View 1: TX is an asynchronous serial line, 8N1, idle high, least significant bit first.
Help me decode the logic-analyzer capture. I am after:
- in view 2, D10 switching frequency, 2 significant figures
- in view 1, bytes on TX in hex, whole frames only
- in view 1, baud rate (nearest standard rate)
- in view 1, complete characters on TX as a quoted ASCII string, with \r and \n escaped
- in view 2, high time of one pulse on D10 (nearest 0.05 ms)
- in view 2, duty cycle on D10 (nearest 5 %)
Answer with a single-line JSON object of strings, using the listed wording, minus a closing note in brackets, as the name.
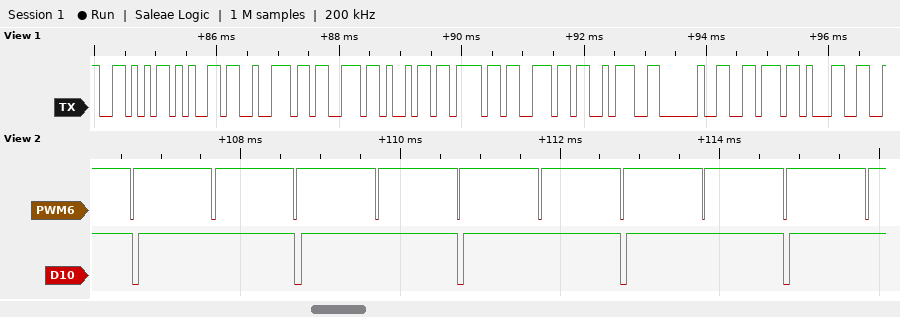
{"in view 2, D10 switching frequency, 2 significant figures": "490 Hz", "in view 1, bytes on TX in hex, whole frames only": "0x56 0x65 0x72 0x73 0x69 0x6F 0x6E 0x3A 0x20 0x76 0x31", "in view 1, baud rate": "9600 baud", "in view 1, complete characters on TX as a quoted ASCII string, with \\r and \\n escaped": "\"Version: v1\"", "in view 2, high time of one pulse on D10": "1.95 ms", "in view 2, duty cycle on D10": "95 %"}
